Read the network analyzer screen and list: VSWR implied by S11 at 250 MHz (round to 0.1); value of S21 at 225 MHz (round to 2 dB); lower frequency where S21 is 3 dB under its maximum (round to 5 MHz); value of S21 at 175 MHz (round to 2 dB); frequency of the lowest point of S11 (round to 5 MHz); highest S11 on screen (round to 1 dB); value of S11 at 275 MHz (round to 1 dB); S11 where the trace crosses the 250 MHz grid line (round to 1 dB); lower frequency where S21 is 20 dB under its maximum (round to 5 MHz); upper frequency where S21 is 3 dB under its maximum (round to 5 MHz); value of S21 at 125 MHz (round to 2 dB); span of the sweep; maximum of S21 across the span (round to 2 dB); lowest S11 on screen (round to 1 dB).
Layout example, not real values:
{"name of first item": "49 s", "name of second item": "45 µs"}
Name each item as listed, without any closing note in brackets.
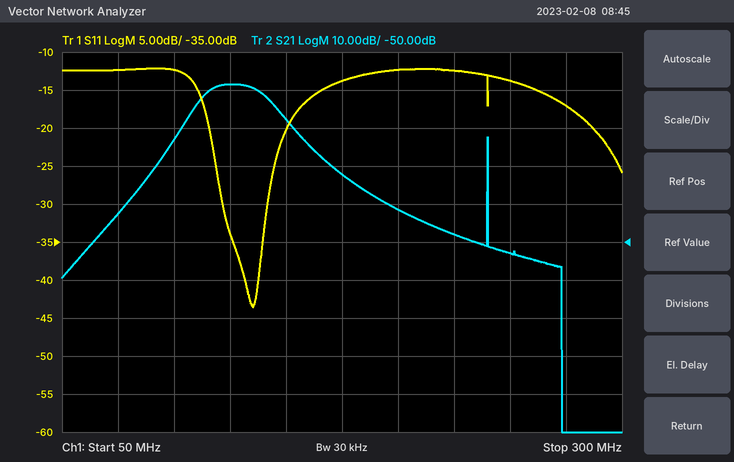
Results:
{"VSWR implied by S11 at 250 MHz": "1.5", "value of S21 at 225 MHz": "-48 dB", "lower frequency where S21 is 3 dB under its maximum": "115 MHz", "value of S21 at 175 MHz": "-32 dB", "frequency of the lowest point of S11": "135 MHz", "highest S11 on screen": "-12 dB", "value of S11 at 275 MHz": "-17 dB", "S11 where the trace crosses the 250 MHz grid line": "-14 dB", "lower frequency where S21 is 20 dB under its maximum": "95 MHz", "upper frequency where S21 is 3 dB under its maximum": "140 MHz", "value of S21 at 125 MHz": "-8 dB", "span of the sweep": "250 MHz", "maximum of S21 across the span": "-8 dB", "lowest S11 on screen": "-44 dB"}
